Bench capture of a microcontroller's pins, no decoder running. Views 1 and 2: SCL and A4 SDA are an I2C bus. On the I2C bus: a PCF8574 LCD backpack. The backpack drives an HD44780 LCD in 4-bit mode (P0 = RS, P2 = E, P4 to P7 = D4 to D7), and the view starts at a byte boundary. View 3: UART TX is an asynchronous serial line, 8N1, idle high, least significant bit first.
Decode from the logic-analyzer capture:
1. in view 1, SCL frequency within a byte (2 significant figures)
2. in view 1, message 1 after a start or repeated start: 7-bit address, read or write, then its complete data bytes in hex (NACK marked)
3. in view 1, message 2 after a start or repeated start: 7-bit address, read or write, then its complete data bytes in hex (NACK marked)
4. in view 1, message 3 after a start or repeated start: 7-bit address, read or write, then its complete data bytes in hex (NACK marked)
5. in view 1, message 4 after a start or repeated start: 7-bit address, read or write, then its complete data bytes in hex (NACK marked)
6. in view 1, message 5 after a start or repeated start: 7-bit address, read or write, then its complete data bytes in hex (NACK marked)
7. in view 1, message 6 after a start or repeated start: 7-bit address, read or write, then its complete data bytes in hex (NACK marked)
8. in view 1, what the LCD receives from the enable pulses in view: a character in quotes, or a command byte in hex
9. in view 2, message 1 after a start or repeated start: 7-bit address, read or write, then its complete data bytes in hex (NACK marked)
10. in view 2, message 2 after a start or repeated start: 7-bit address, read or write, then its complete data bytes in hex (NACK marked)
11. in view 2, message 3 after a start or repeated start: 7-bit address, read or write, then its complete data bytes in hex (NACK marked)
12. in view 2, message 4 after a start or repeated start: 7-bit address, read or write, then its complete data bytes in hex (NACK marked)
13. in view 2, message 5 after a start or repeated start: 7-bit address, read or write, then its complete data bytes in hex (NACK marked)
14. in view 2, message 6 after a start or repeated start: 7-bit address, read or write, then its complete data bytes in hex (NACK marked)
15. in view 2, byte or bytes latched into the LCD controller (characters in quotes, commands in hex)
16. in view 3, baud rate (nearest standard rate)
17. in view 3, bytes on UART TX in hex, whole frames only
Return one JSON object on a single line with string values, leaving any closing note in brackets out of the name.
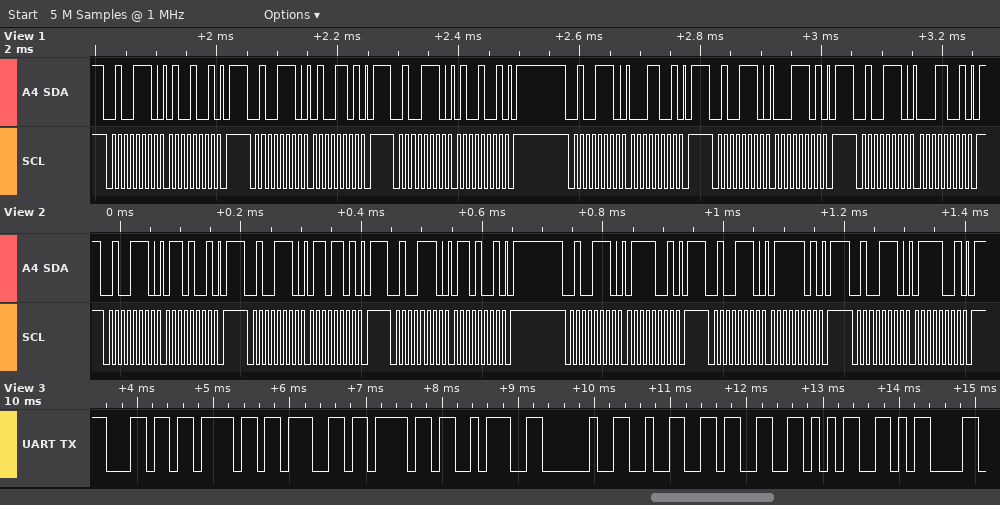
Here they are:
{"in view 1, SCL frequency within a byte": "100 kHz", "in view 1, message 1 after a start or repeated start: 7-bit address, read or write, then its complete data bytes in hex": "0x27 write: 49", "in view 1, message 2 after a start or repeated start: 7-bit address, read or write, then its complete data bytes in hex": "0x27 write: 4D", "in view 1, message 3 after a start or repeated start: 7-bit address, read or write, then its complete data bytes in hex": "0x27 write: 49", "in view 1, message 4 after a start or repeated start: 7-bit address, read or write, then its complete data bytes in hex": "0x27 write: 19", "in view 1, message 5 after a start or repeated start: 7-bit address, read or write, then its complete data bytes in hex": "0x27 write: 1D", "in view 1, message 6 after a start or repeated start: 7-bit address, read or write, then its complete data bytes in hex": "0x27 write: 19", "in view 1, what the LCD receives from the enable pulses in view: a character in quotes, or a command byte in hex": "'A'", "in view 2, message 1 after a start or repeated start: 7-bit address, read or write, then its complete data bytes in hex": "0x27 write: 69", "in view 2, message 2 after a start or repeated start: 7-bit address, read or write, then its complete data bytes in hex": "0x27 write: 6D", "in view 2, message 3 after a start or repeated start: 7-bit address, read or write, then its complete data bytes in hex": "0x27 write: 69", "in view 2, message 4 after a start or repeated start: 7-bit address, read or write, then its complete data bytes in hex": "0x27 write: 79", "in view 2, message 5 after a start or repeated start: 7-bit address, read or write, then its complete data bytes in hex": "0x27 write: 7D", "in view 2, message 6 after a start or repeated start: 7-bit address, read or write, then its complete data bytes in hex": "0x27 write: 79", "in view 2, byte or bytes latched into the LCD controller": "'g'", "in view 3, baud rate": "9600 baud", "in view 3, bytes on UART TX in hex, whole frames only": "0x6C 0x6F 0x67 0x6F 0x3A 0x20 0x32 0x33 0x35 0x0D"}
